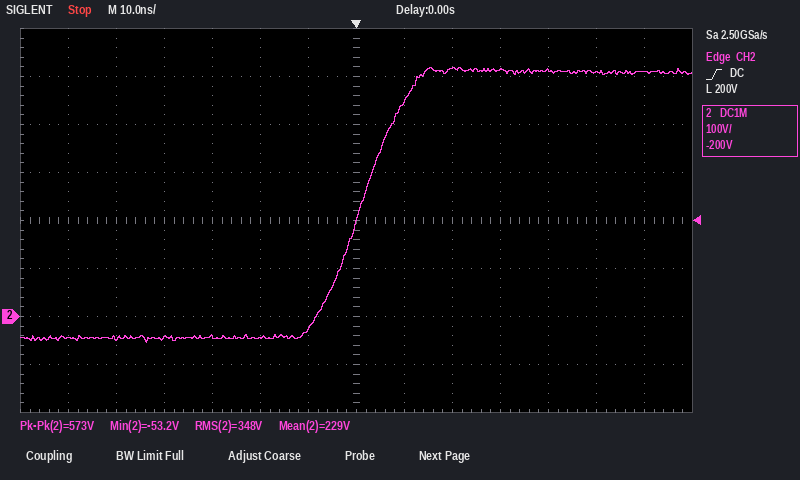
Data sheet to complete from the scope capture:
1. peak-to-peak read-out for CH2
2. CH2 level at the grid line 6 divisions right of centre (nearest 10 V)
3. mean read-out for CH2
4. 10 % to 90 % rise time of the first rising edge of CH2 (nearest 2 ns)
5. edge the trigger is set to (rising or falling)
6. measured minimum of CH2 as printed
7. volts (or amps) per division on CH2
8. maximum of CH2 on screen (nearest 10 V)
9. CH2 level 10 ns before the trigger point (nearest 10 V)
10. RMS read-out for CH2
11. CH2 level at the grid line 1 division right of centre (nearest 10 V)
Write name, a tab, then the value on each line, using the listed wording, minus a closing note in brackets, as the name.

peak-to-peak read-out for CH2	573 V
CH2 level at the grid line 6 divisions right of centre	510 V
mean read-out for CH2	229 V
10 % to 90 % rise time of the first rising edge of CH2	18 ns
edge the trigger is set to	rising
measured minimum of CH2 as printed	-53.2 V
volts (or amps) per division on CH2	100 V
maximum of CH2 on screen	520 V
CH2 level 10 ns before the trigger point	-30 V
RMS read-out for CH2	348 V
CH2 level at the grid line 1 division right of centre	450 V
